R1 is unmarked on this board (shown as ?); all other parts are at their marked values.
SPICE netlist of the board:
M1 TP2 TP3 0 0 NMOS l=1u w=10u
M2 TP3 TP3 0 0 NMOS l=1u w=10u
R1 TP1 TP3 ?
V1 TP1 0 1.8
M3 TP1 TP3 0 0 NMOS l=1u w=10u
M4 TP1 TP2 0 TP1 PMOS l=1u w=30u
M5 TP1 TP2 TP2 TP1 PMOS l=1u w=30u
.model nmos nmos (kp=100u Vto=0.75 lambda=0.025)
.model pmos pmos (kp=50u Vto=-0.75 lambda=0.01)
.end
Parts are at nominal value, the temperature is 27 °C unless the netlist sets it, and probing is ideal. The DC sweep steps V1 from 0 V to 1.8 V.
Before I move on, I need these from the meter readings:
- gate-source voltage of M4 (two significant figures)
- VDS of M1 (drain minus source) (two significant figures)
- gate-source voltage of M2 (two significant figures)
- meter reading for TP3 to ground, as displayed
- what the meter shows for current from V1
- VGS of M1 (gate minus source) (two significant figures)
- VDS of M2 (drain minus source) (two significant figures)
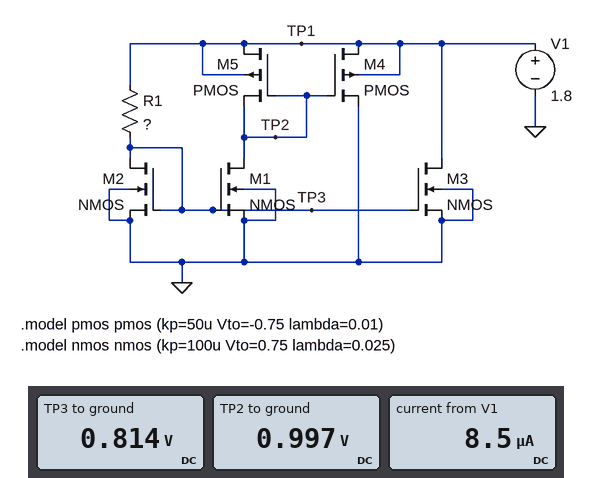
1.0 V
1.0 V
810 mV
0.814 V
8.5 µA
810 mV
810 mV
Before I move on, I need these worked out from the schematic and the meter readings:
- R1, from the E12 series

470 kΩ
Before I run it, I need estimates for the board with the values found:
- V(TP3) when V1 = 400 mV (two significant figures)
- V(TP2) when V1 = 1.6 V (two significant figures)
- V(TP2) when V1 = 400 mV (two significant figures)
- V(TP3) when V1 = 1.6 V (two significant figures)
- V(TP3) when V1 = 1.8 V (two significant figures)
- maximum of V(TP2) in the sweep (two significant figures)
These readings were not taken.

400 mV
800 mV
200 mV
810 mV
810 mV
1.0 V
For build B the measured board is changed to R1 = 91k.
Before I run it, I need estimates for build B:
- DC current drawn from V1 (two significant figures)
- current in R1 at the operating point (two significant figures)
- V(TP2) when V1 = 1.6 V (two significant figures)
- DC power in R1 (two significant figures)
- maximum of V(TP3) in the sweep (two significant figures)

40 µA
10 µA
750 mV
9.1 µW
890 mV
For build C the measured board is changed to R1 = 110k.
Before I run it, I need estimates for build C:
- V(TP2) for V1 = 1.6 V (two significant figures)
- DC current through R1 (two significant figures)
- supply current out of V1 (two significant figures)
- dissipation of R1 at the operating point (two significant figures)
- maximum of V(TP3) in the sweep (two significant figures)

760 mV
8.4 µA
34 µA
7.7 µW
880 mV
